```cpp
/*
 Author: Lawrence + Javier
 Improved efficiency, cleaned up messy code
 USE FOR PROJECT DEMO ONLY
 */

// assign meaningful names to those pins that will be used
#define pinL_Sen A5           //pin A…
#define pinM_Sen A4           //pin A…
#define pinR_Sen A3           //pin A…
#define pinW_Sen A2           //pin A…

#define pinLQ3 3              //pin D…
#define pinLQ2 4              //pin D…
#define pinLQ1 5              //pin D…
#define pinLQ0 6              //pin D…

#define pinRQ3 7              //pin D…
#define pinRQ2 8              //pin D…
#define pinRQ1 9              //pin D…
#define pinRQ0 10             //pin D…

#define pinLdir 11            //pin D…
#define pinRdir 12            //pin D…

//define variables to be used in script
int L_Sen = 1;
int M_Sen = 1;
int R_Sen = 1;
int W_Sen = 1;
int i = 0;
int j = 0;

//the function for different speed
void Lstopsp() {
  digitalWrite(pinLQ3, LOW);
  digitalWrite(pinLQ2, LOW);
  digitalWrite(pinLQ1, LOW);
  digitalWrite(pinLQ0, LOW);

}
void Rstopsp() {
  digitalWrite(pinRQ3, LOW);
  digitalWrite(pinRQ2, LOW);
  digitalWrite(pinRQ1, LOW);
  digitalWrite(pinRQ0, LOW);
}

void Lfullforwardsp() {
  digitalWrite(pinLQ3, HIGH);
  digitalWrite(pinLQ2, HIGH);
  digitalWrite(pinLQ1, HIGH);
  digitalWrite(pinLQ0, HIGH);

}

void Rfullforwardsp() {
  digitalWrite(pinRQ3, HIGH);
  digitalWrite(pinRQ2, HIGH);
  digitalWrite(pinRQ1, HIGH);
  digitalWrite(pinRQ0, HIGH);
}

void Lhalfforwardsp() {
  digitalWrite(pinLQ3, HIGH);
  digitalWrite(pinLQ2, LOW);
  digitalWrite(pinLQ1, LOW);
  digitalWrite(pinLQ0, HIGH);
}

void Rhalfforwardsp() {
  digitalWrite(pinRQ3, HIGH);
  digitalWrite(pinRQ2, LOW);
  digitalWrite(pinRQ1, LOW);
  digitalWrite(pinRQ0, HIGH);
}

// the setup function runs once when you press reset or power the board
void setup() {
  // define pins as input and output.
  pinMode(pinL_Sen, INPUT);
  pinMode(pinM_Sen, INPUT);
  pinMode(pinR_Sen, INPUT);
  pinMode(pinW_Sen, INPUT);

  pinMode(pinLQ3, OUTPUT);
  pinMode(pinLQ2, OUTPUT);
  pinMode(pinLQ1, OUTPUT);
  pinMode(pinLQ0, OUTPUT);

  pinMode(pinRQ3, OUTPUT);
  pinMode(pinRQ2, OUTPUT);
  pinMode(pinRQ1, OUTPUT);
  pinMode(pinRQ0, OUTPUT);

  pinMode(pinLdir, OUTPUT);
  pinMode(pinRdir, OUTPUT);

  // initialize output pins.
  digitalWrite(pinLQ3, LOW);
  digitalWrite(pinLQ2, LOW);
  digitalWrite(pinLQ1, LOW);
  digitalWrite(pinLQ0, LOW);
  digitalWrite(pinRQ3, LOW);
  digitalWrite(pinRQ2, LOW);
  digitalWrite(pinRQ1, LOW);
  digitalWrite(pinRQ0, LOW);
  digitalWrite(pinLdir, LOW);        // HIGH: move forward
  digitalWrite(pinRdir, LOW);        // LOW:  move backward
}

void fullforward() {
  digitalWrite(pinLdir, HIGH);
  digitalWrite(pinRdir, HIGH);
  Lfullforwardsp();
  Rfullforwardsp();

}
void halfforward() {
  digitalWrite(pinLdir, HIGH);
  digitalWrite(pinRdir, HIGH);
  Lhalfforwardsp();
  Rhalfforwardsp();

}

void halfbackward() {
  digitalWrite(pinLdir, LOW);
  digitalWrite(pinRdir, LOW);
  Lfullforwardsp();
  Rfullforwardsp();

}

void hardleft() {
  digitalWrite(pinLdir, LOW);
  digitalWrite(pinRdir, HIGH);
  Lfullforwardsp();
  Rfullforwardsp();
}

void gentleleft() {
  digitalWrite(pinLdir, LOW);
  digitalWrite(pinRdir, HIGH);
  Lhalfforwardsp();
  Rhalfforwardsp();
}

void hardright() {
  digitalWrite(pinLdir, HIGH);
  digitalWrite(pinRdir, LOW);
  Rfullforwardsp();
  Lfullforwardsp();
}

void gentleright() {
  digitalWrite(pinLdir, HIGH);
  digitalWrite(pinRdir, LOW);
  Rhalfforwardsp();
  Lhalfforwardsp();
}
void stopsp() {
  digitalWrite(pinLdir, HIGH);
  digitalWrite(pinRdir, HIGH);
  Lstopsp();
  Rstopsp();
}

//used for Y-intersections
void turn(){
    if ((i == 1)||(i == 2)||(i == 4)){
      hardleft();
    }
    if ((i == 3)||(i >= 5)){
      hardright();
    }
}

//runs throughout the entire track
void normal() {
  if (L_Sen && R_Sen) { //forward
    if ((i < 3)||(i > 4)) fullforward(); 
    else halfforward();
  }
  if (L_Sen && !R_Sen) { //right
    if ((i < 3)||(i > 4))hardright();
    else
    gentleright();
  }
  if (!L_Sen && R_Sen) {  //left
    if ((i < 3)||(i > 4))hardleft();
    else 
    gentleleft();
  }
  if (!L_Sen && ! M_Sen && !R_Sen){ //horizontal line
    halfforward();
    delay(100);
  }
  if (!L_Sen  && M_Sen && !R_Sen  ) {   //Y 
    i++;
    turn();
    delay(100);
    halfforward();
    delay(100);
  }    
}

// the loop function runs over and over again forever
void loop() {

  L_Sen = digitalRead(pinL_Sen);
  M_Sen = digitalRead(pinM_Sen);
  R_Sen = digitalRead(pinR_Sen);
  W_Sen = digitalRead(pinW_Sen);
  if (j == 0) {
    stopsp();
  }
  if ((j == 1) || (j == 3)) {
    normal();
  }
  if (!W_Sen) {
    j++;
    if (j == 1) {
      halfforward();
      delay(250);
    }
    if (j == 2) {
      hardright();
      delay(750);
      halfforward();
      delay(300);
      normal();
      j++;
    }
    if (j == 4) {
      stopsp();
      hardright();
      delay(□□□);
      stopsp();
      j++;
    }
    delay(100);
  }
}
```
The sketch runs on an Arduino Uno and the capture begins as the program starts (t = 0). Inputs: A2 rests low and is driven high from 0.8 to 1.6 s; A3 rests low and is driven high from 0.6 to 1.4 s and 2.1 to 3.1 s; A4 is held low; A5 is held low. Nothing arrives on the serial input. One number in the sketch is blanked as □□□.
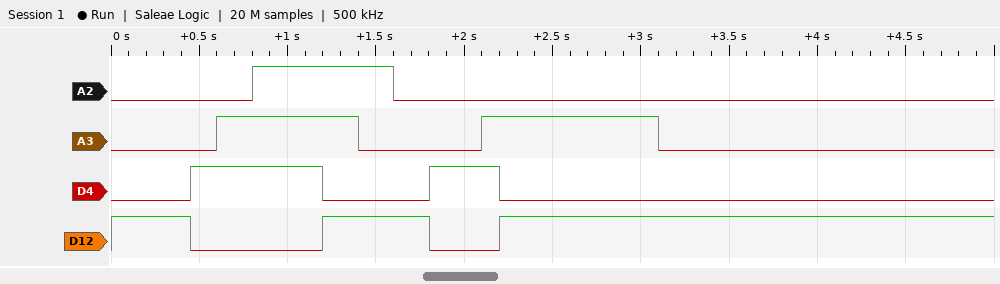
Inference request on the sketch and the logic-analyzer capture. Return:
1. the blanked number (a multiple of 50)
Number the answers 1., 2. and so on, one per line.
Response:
1. 400
